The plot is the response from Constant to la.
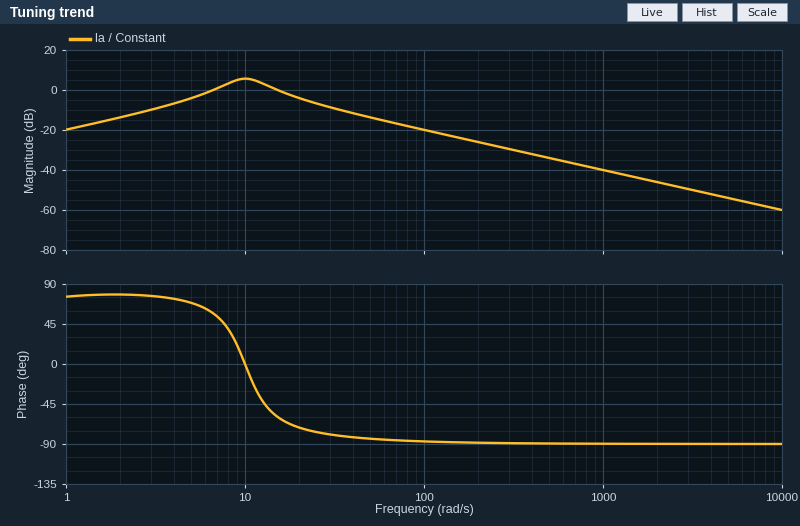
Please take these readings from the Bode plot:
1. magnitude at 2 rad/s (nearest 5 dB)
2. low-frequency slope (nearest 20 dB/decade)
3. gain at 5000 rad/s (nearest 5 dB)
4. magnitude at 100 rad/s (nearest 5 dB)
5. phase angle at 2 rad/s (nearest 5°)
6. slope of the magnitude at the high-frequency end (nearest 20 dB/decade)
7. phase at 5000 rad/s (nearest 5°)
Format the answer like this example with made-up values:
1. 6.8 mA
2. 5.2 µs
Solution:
1. -15 dB
2. 20 dB/decade
3. -55 dB
4. -20 dB
5. 80°
6. -20 dB/decade
7. -90°
